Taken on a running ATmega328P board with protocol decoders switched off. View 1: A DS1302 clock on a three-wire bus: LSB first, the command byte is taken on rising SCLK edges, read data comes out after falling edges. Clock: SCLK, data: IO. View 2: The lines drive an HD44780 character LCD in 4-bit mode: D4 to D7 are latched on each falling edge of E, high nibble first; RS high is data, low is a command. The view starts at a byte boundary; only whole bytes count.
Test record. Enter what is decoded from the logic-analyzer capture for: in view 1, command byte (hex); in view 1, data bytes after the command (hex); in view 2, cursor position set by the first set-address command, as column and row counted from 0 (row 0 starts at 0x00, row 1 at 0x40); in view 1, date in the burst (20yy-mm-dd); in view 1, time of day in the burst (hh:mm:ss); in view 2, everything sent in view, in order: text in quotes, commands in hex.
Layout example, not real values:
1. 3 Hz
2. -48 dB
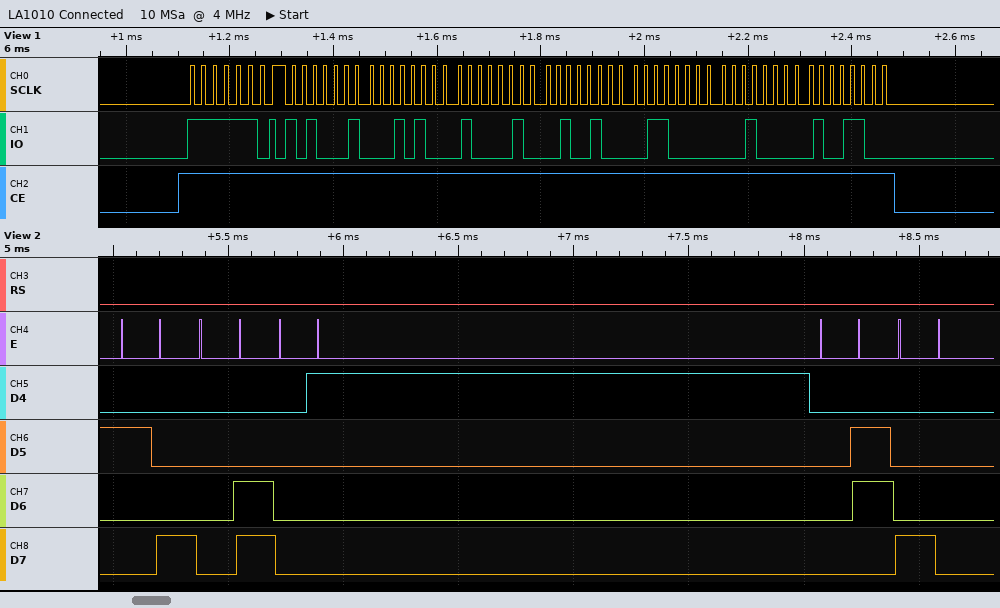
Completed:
1. 0xBF
2. 45 14 21 12 06 04 19
3. column 0, row 0
4. 2019-06-12
5. 21:14:45
6. 0x28 0x0C 0x01 0x06 0x80
